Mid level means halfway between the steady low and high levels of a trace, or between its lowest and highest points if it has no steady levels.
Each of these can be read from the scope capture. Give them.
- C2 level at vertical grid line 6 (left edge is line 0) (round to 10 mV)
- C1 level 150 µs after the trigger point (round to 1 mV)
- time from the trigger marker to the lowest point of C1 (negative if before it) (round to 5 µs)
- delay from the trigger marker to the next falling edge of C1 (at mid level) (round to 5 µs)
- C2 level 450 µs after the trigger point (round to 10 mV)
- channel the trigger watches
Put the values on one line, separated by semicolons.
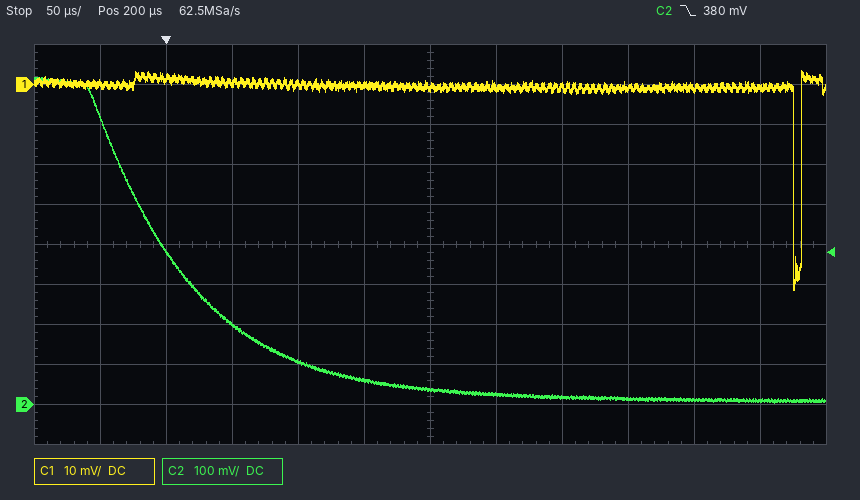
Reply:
40 mV; 0 mV; +475 µs; 475 µs; 10 mV; C2
